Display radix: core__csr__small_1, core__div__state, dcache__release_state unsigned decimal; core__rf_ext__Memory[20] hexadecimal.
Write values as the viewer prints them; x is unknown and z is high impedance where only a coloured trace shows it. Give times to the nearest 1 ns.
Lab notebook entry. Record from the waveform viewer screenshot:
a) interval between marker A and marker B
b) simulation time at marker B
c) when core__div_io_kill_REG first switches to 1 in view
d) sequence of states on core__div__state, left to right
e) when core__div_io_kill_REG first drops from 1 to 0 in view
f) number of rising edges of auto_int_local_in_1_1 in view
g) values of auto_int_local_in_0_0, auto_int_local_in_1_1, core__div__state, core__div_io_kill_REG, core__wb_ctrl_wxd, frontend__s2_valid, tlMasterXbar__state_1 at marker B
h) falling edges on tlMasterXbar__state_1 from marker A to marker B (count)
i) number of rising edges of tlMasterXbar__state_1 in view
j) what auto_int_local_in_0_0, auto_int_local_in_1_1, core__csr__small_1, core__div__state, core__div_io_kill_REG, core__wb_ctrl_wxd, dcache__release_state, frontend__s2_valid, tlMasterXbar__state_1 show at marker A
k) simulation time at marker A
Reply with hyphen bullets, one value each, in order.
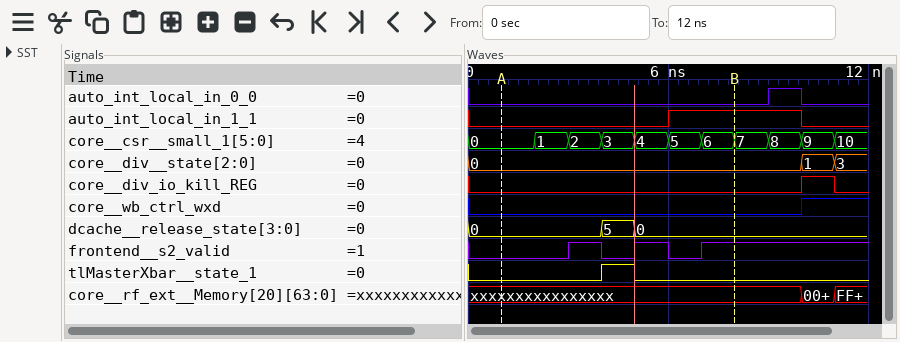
- 7 ns
- 8 ns
- 10 ns
- 0, 1, 3
- 11 ns
- 1
- auto_int_local_in_0_0=0, auto_int_local_in_1_1=1, core__div__state=0, core__div_io_kill_REG=0, core__wb_ctrl_wxd=0, frontend__s2_valid=1, tlMasterXbar__state_1=0
- 1
- 1
- auto_int_local_in_0_0=0, auto_int_local_in_1_1=0, core__csr__small_1=0, core__div__state=0, core__div_io_kill_REG=0, core__wb_ctrl_wxd=0, dcache__release_state=0, frontend__s2_valid=0, tlMasterXbar__state_1=0
- 1 ns
